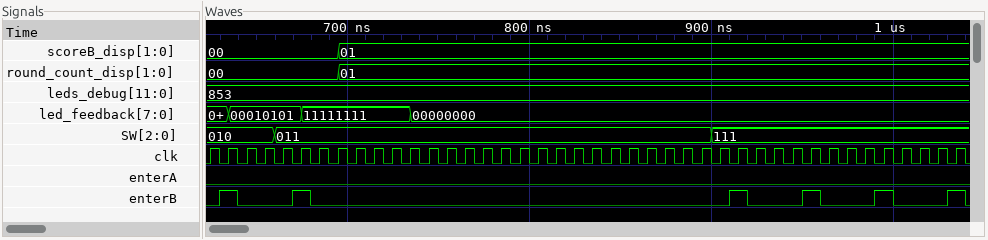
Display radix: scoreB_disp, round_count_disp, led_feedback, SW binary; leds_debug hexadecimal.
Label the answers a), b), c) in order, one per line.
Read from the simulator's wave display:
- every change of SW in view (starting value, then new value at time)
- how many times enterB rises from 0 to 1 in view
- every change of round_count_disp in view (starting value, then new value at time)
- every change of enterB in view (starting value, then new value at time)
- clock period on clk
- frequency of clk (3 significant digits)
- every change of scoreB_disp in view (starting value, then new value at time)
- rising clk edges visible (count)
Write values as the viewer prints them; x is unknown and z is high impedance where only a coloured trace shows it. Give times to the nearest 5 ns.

a) 010, 011 at 660 ns, 111 at 900 ns
b) 6
c) 00, 01 at 695 ns
d) 0, 1 at 630 ns, 0 at 640 ns, 1 at 670 ns, 0 at 680 ns, 1 at 910 ns, 0 at 920 ns, 1 at 950 ns, 0 at 960 ns, 1 at 990 ns, 0 at 1000 ns, 1 at 1030 ns, 0 at 1040 ns
e) 10 ns
f) 100 MHz
g) 00, 01 at 695 ns
h) 42
